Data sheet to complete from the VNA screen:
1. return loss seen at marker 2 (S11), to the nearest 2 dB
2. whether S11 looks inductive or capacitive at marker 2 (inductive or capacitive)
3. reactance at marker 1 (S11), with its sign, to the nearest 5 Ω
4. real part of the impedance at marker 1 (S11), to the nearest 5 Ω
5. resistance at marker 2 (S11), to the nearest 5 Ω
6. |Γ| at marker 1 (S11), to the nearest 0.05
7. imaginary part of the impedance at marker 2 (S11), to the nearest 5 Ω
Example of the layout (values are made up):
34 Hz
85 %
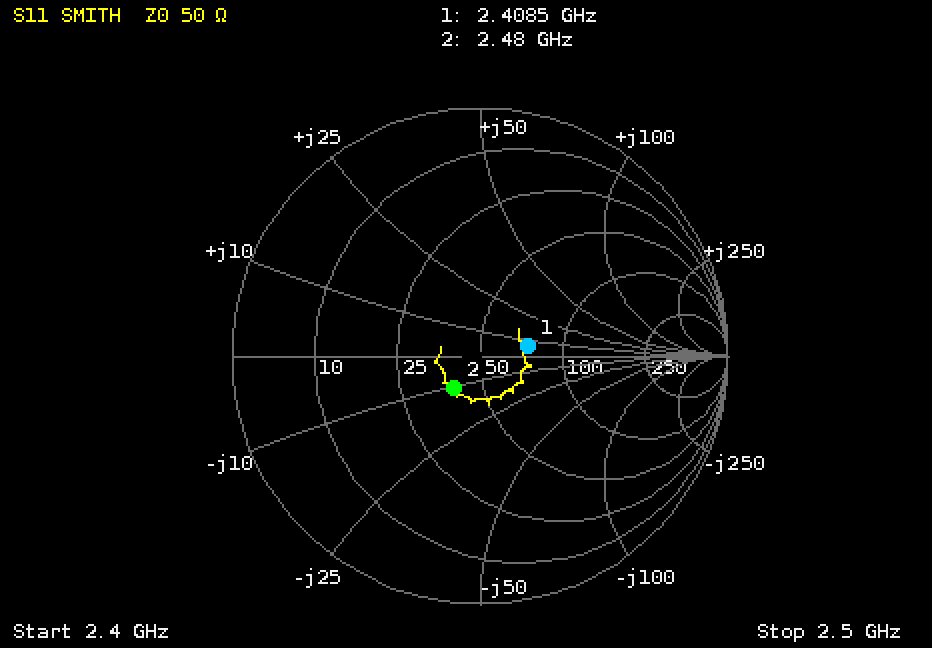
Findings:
16 dB
capacitive
+5 Ω
75 Ω
40 Ω
0.20
-10 Ω
